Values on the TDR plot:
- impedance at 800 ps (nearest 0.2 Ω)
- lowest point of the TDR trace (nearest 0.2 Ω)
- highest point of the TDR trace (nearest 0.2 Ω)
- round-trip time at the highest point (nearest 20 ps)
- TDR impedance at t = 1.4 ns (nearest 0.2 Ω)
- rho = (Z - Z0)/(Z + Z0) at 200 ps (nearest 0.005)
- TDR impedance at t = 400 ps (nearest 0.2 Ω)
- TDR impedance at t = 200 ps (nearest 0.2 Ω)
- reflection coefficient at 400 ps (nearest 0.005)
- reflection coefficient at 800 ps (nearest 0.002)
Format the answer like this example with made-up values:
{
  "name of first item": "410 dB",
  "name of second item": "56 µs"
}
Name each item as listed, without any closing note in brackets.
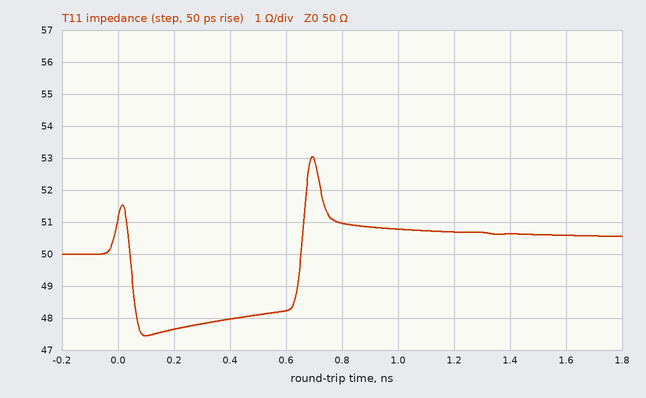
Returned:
{
  "impedance at 800 ps": "51.0 Ω",
  "lowest point of the TDR trace": "47.4 Ω",
  "highest point of the TDR trace": "53.0 Ω",
  "round-trip time at the highest point": "700 ps",
  "TDR impedance at t = 1.4 ns": "50.6 Ω",
  "rho = (Z - Z0)/(Z + Z0) at 200 ps": "-0.025",
  "TDR impedance at t = 400 ps": "48.0 Ω",
  "TDR impedance at t = 200 ps": "47.6 Ω",
  "reflection coefficient at 400 ps": "-0.020",
  "reflection coefficient at 800 ps": "+0.010"
}
